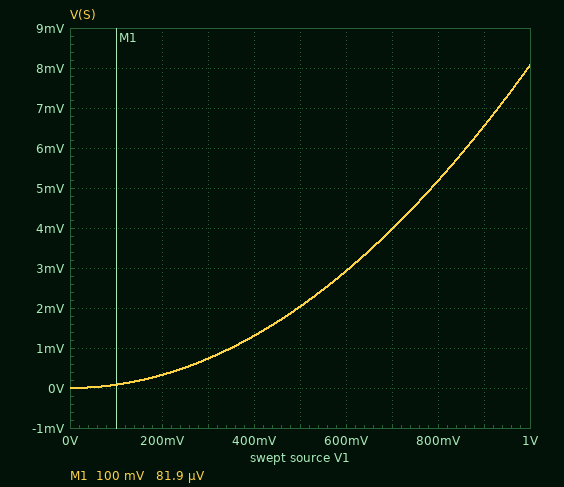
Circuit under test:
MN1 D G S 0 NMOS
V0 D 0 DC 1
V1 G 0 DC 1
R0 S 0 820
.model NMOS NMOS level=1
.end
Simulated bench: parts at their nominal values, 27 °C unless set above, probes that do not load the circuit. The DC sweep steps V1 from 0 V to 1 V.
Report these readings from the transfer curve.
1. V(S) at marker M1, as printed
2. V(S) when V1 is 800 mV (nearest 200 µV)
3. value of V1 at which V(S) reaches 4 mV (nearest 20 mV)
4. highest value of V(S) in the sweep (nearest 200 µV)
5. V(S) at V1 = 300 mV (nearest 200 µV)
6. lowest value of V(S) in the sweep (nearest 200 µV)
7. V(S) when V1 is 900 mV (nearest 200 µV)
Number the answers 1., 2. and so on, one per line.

1. 81.9 µV
2. 5.2 mV
3. 700 mV
4. 8.0 mV
5. 800 µV
6. 0 V
7. 6.6 mV
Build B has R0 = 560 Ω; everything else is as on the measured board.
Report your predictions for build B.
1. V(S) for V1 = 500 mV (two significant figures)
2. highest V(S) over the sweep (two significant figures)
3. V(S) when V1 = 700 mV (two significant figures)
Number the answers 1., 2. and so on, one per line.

1. 1.4 mV
2. 5.5 mV
3. 2.7 mV
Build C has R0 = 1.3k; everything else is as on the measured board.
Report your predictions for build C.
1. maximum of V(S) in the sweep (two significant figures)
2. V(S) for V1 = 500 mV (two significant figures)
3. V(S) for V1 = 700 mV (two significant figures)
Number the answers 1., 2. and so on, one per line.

1. 13 mV
2. 3.2 mV
3. 6.3 mV
